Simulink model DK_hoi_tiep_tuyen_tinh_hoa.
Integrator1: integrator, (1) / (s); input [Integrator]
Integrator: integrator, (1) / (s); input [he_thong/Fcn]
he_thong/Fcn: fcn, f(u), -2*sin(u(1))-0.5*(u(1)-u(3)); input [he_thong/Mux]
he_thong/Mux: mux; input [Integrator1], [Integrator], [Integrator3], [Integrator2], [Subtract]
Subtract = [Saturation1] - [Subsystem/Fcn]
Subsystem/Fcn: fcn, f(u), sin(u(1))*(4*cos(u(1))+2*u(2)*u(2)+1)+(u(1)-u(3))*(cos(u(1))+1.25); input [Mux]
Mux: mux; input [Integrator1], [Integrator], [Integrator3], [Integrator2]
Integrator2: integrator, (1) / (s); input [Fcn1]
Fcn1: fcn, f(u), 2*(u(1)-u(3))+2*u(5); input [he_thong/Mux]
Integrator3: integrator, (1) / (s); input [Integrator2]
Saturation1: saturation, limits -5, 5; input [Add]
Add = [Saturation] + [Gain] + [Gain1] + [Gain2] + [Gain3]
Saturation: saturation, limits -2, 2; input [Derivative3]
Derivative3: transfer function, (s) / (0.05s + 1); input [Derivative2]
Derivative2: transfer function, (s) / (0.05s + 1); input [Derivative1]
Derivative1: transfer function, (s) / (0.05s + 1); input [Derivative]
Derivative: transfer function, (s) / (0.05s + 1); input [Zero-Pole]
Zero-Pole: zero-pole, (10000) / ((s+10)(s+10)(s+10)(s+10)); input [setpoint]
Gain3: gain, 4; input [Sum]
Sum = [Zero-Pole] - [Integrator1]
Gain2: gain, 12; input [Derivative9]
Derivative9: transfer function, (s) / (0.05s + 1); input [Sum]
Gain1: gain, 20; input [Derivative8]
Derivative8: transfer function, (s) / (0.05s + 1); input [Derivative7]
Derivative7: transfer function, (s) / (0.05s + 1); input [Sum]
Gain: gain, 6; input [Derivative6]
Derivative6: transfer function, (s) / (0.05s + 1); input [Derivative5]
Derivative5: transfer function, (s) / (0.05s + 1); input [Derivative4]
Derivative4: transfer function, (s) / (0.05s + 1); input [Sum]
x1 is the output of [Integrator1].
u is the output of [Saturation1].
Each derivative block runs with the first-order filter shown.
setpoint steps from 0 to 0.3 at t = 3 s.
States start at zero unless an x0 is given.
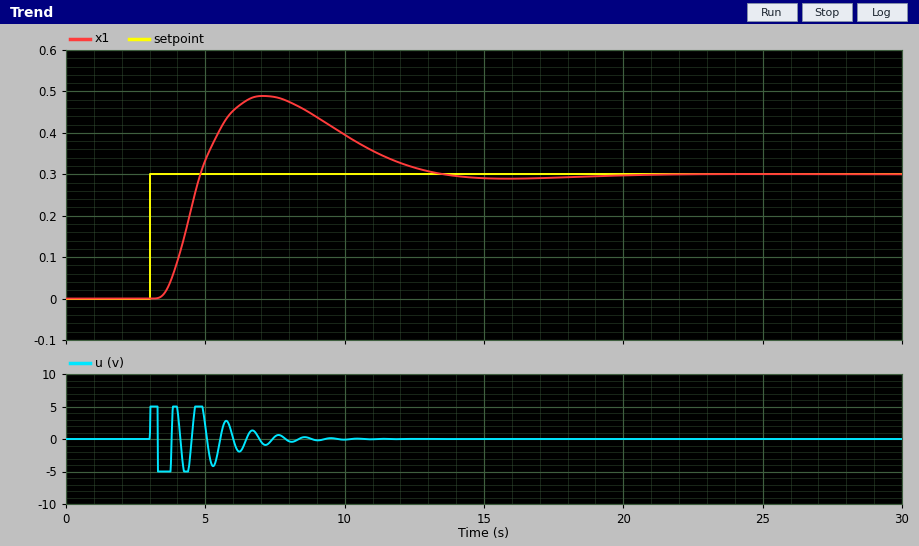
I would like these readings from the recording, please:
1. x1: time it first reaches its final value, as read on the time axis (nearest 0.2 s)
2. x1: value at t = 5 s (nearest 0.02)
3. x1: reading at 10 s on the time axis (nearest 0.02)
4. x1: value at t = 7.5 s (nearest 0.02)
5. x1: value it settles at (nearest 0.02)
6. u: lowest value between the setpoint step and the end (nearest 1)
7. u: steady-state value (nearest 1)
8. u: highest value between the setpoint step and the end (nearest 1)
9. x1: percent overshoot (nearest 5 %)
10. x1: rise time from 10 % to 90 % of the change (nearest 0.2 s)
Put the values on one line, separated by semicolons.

4.8 s; 0.34; 0.40; 0.48; 0.30; -5; 0; 5; 65 %; 1.0 s
